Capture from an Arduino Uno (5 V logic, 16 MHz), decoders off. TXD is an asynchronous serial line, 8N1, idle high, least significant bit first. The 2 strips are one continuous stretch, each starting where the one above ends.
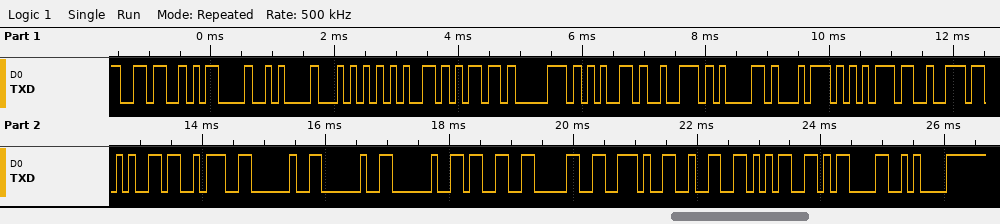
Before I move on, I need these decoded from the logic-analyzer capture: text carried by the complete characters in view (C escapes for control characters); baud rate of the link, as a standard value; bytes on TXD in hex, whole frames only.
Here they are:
"6\r\nTemperature:   30.25\r\n"
9600 baud
36 0D 0A 54 65 6D 70 65 72 61 74 75 72 65 3A 20 20 20 33 30 2E 32 35 0D 0A
